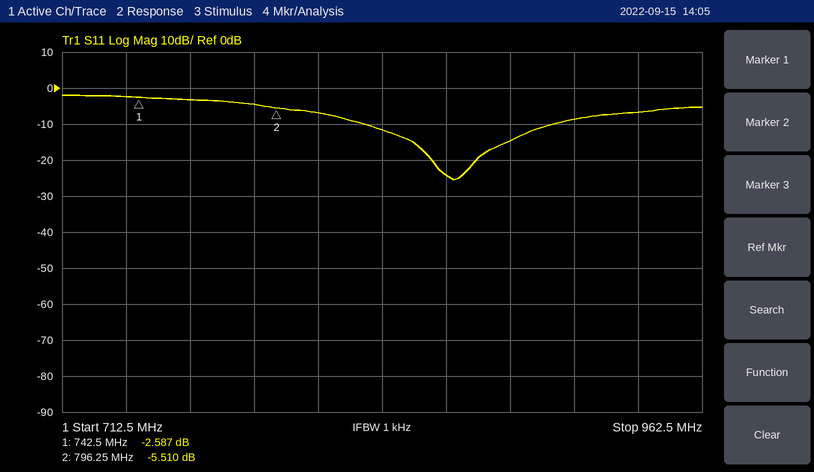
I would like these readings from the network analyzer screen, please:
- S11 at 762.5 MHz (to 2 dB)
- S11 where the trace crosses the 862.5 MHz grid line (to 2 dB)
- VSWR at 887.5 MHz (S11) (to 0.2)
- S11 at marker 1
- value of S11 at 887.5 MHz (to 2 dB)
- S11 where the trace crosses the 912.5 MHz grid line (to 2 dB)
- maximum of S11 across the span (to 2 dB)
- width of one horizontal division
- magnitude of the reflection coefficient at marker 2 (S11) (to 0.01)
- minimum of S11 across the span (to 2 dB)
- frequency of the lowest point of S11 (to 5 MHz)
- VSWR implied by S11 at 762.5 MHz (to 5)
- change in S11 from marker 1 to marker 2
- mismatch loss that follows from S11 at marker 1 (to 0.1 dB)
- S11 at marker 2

-4 dB
-24 dB
1.4
-2.587 dB
-14 dB
-8 dB
-2 dB
25 MHz
0.53
-26 dB
865 MHz
5
-2.923 dB
3.5 dB
-5.510 dB
